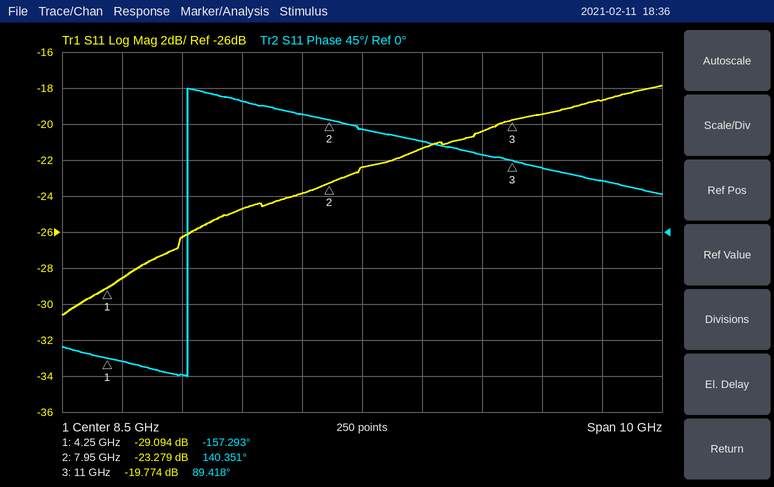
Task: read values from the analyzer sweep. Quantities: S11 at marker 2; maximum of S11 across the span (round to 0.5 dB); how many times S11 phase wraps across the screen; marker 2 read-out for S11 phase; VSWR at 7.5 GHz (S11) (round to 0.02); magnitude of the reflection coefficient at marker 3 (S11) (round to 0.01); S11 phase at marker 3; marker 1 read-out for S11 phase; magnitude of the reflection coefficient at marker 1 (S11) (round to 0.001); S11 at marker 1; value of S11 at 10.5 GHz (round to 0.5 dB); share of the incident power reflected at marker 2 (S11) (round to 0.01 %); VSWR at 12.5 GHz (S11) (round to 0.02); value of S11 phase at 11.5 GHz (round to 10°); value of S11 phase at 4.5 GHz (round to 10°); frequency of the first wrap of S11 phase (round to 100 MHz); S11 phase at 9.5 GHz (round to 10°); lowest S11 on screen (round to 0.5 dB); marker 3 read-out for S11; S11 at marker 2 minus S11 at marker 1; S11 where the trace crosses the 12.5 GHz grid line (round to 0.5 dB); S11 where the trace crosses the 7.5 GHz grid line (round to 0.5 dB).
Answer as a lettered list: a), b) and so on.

a) -23.279 dB
b) -18.0 dB
c) 1
d) 140.351°
e) 1.14
f) 0.10
g) 89.418°
h) -157.293°
i) 0.035
j) -29.094 dB
k) -20.5 dB
l) 0.47 %
m) 1.26
n) 80°
o) -160°
p) 5.6 GHz
q) 110°
r) -30.5 dB
s) -19.774 dB
t) 5.815 dB
u) -18.5 dB
v) -24.0 dB
